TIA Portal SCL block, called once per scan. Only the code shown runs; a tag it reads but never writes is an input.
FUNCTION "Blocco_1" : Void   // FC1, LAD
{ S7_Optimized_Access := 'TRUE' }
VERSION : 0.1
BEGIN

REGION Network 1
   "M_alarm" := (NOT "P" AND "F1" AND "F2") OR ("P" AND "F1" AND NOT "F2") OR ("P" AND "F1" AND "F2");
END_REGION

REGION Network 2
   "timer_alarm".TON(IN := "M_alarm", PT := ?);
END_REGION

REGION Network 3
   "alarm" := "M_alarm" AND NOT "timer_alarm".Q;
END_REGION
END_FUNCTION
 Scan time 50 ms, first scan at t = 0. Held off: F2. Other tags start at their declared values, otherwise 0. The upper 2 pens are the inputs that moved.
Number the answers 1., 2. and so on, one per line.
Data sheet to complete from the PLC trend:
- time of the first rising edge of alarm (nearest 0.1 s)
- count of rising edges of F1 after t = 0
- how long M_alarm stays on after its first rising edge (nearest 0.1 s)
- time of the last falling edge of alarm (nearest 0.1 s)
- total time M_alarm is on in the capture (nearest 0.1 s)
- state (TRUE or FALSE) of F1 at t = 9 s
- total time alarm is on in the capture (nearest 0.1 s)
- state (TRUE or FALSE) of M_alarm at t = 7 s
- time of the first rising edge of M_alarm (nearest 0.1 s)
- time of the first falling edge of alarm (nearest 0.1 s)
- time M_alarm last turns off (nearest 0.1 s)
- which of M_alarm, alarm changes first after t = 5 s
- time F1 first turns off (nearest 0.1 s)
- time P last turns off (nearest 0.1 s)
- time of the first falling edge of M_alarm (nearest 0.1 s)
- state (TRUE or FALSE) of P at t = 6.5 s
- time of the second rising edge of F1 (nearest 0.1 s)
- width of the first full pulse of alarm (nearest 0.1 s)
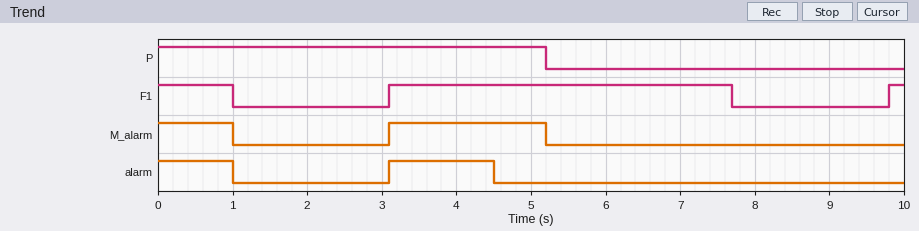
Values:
1. 3.1 s
2. 2
3. 2.1 s
4. 4.5 s
5. 3.1 s
6. FALSE
7. 2.4 s
8. FALSE
9. 3.1 s
10. 1.0 s
11. 5.2 s
12. M_alarm
13. 1.0 s
14. 5.2 s
15. 1.0 s
16. FALSE
17. 9.8 s
18. 1.4 s
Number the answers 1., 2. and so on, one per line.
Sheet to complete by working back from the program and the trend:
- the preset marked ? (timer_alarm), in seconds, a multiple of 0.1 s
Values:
1. 1.4 s
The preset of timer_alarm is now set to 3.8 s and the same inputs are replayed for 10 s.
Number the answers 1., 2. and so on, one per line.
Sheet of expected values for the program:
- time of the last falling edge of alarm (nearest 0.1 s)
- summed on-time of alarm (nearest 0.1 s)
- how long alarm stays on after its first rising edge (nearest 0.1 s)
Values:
1. 5.2 s
2. 3.1 s
3. 2.1 s
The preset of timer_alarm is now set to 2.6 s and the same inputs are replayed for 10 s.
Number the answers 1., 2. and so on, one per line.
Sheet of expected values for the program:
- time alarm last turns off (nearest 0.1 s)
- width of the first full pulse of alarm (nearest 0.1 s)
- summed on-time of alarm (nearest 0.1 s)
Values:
1. 5.2 s
2. 2.1 s
3. 3.1 s
